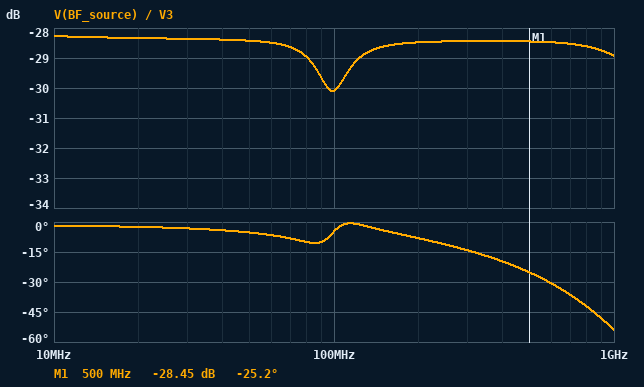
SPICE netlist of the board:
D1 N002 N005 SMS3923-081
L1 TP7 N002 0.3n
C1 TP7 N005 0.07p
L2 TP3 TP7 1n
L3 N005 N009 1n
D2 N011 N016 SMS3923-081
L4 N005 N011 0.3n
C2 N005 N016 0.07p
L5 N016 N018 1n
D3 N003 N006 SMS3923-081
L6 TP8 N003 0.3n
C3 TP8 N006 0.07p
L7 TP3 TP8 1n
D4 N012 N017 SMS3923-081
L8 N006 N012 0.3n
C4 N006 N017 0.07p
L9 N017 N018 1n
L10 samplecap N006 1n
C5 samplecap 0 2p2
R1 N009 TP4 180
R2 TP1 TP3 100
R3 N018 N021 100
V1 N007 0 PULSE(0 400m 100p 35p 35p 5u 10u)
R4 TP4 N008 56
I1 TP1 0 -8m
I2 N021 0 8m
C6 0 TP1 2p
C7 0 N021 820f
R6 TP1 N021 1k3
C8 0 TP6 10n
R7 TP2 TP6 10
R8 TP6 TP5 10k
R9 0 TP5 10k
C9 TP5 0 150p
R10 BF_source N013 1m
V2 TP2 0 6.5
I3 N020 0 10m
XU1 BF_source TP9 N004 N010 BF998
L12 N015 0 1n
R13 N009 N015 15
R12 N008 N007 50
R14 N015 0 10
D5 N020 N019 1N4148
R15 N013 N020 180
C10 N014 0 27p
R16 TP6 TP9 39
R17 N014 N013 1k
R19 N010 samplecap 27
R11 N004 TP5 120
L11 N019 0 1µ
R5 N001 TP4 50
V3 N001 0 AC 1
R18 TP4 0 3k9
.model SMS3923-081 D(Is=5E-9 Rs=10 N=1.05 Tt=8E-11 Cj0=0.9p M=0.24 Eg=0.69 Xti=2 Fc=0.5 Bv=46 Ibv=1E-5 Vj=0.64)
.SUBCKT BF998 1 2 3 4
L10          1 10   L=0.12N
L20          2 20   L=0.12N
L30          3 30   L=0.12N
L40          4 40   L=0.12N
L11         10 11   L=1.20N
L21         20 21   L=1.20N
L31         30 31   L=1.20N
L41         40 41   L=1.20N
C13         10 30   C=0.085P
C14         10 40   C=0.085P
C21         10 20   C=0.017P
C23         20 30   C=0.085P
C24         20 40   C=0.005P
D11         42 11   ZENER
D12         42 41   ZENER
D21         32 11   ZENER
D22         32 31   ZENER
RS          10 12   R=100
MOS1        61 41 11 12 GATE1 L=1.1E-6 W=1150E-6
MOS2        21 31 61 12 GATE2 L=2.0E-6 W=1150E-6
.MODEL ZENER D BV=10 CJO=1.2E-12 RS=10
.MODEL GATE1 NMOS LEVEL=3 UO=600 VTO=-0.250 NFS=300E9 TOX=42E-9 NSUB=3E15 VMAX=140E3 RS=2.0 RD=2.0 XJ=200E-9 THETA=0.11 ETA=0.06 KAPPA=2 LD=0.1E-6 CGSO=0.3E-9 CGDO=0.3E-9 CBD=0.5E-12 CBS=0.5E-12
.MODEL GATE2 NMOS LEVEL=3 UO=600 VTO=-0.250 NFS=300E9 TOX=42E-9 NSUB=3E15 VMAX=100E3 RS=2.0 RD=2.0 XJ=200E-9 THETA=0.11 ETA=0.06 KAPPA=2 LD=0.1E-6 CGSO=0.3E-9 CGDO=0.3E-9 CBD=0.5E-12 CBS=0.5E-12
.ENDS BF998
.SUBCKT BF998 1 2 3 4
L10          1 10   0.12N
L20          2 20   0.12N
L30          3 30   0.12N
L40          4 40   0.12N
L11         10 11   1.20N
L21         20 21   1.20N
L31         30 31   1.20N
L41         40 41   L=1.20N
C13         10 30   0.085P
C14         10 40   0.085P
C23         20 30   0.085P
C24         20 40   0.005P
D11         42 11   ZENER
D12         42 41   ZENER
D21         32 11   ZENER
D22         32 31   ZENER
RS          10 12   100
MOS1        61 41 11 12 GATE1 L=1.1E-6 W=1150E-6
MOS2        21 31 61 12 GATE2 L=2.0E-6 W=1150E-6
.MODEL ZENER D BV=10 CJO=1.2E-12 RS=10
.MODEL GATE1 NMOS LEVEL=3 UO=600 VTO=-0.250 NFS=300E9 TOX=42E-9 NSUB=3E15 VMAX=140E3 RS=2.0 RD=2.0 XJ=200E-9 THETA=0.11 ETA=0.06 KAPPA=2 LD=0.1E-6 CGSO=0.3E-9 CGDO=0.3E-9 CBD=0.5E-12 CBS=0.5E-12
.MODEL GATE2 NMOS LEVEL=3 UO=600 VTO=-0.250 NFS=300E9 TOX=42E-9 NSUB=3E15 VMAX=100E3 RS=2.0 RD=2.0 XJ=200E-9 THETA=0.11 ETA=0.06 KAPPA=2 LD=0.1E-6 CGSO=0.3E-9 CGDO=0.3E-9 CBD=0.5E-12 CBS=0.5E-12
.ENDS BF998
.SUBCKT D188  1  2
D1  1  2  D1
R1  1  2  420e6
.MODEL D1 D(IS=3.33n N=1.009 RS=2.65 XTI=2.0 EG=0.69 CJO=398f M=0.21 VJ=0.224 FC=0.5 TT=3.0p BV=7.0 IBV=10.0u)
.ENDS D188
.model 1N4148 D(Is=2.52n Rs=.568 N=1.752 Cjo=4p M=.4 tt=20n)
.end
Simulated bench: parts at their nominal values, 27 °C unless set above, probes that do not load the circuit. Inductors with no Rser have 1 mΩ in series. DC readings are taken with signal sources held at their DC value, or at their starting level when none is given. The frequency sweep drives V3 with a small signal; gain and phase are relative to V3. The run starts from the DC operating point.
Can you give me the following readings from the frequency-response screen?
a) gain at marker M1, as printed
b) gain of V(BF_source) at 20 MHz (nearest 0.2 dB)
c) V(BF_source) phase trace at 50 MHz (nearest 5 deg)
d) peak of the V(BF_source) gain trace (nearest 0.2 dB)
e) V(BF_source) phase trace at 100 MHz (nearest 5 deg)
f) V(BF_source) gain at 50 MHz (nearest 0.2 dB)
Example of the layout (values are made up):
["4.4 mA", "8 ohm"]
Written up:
["-28.45 dB", "-28.4 dB", "-5 deg", "-28.2 dB", "-5 deg", "-28.4 dB"]
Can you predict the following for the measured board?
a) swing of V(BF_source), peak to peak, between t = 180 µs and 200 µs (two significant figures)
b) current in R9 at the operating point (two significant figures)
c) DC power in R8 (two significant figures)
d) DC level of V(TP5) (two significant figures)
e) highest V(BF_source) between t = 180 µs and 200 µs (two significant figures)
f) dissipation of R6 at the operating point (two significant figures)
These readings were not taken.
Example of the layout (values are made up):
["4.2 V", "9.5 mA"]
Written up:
["7.5 mV", "320 µA", "1.0 mW", "3.2 V", "-100 mV", "3.3 mW"]
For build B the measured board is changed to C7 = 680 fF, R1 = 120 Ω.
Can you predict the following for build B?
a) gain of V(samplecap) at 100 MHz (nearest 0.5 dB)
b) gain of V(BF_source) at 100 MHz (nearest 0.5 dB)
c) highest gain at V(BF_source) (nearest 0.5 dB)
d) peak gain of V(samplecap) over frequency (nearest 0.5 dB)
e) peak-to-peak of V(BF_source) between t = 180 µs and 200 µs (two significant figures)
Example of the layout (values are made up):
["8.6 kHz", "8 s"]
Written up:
["-24.5 dB", "-27.5 dB", "-25.5 dB", "-24.0 dB", "10 mV"]
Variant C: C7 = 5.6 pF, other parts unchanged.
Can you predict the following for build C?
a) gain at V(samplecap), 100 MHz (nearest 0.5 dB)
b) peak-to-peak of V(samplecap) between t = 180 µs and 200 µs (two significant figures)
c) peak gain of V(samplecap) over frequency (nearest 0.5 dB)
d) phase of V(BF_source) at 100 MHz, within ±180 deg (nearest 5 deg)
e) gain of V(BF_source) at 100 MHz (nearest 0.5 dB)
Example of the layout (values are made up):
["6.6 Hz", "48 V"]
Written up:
["-27.5 dB", "8.4 mV", "-27.0 dB", "-10 deg", "-30.5 dB"]
